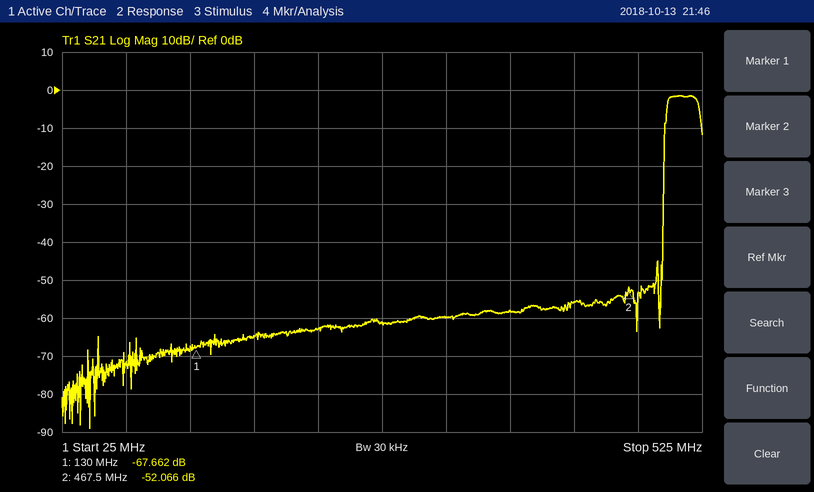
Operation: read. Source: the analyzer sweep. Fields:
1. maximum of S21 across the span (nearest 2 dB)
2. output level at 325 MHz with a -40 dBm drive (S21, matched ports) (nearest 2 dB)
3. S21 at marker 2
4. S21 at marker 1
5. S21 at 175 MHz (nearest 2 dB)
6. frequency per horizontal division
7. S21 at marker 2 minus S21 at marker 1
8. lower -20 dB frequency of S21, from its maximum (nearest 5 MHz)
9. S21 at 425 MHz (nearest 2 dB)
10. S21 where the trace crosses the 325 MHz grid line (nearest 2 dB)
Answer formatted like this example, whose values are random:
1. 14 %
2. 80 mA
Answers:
1. -2 dB
2. -100 dBm
3. -52.066 dB
4. -67.662 dB
5. -64 dB
6. 50 MHz
7. 15.596 dB
8. 495 MHz
9. -56 dB
10. -60 dB
